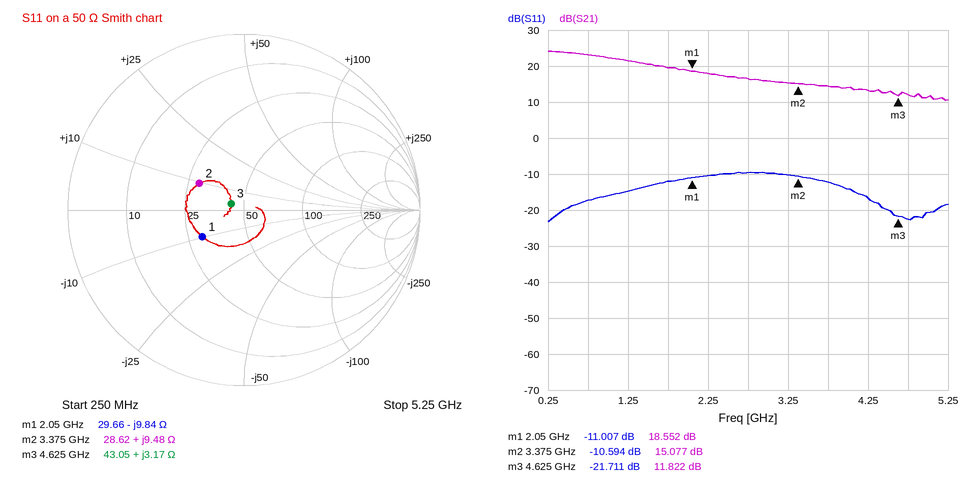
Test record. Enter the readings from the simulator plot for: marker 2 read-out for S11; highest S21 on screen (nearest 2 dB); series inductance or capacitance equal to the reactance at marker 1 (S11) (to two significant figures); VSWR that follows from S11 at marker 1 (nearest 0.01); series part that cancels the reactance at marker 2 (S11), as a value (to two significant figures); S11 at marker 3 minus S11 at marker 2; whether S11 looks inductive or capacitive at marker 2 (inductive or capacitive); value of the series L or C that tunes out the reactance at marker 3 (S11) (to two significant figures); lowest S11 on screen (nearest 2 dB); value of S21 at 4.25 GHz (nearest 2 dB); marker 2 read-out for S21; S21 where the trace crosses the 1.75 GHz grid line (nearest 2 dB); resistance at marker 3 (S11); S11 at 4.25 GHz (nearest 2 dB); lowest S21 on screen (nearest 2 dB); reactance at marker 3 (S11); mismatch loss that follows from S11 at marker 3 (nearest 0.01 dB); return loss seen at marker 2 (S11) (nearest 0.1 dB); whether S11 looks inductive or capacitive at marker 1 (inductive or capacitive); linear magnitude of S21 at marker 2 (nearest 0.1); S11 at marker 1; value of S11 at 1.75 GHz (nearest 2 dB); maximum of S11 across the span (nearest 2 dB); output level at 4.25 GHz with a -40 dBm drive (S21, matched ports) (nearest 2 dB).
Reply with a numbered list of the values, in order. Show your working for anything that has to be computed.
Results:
1. -10.594 dB
2. 24 dB
3. C = 1/(2π × 2.05 GHz × 9.84 Ω) ≈ 7.9 pF
4. (1 + 0.2816)/(1 − 0.2816) ≈ 1.78
5. C = 1/(2π × 3.375 GHz × 9.48 Ω) ≈ 5.0 pF
6. -21.711 − (-10.594) = -11.117 dB
7. inductive
8. C = 1/(2π × 4.625 GHz × 3.17 Ω) ≈ 11 pF
9. -24 dB
10. 14 dB
11. 15.077 dB
12. 20 dB
13. 43.05 Ω
14. -16 dB
15. 10 dB
16. +3.17 Ω
17. −10 log10(1 − 10^(-21.711/10)) ≈ 0.03 dB
18. 10.6 dB
19. capacitive
20. 10^(15.077/20) ≈ 5.7
21. -11.007 dB
22. -12 dB
23. -10 dB
24. -40 dBm + (14 dB) = -26 dBm
